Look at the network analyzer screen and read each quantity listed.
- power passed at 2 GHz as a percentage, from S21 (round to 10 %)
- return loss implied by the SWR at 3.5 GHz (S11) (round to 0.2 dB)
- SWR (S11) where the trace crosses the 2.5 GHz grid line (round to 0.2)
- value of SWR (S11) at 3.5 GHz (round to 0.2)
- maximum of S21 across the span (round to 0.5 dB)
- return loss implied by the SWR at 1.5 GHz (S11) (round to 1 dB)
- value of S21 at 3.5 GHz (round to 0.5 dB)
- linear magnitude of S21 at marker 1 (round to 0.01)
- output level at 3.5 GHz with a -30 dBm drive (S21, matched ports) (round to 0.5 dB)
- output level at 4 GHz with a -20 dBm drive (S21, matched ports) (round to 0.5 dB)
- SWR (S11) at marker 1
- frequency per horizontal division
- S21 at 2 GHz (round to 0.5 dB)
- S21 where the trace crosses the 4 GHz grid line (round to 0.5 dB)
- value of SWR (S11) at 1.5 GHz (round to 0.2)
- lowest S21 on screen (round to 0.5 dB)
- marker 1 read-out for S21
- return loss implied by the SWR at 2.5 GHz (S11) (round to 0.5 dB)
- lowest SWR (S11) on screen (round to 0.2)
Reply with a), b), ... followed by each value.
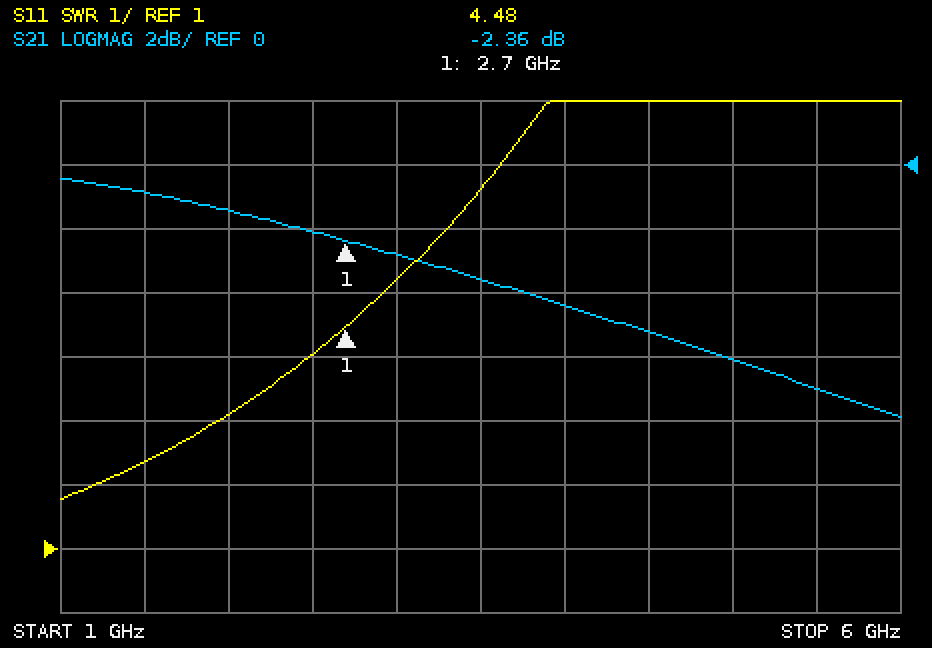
a) 70 %
b) 2.6 dB
c) 4.0
d) 6.6
e) -0.5 dB
f) 8 dB
g) -3.5 dB
h) 0.76
i) -33.5 dBm
j) -24.5 dBm
k) 4.48
l) 500 MHz
m) -1.5 dB
n) -4.5 dB
o) 2.4
p) -8.0 dB
q) -2.36 dB
r) 4.5 dB
s) 1.8
